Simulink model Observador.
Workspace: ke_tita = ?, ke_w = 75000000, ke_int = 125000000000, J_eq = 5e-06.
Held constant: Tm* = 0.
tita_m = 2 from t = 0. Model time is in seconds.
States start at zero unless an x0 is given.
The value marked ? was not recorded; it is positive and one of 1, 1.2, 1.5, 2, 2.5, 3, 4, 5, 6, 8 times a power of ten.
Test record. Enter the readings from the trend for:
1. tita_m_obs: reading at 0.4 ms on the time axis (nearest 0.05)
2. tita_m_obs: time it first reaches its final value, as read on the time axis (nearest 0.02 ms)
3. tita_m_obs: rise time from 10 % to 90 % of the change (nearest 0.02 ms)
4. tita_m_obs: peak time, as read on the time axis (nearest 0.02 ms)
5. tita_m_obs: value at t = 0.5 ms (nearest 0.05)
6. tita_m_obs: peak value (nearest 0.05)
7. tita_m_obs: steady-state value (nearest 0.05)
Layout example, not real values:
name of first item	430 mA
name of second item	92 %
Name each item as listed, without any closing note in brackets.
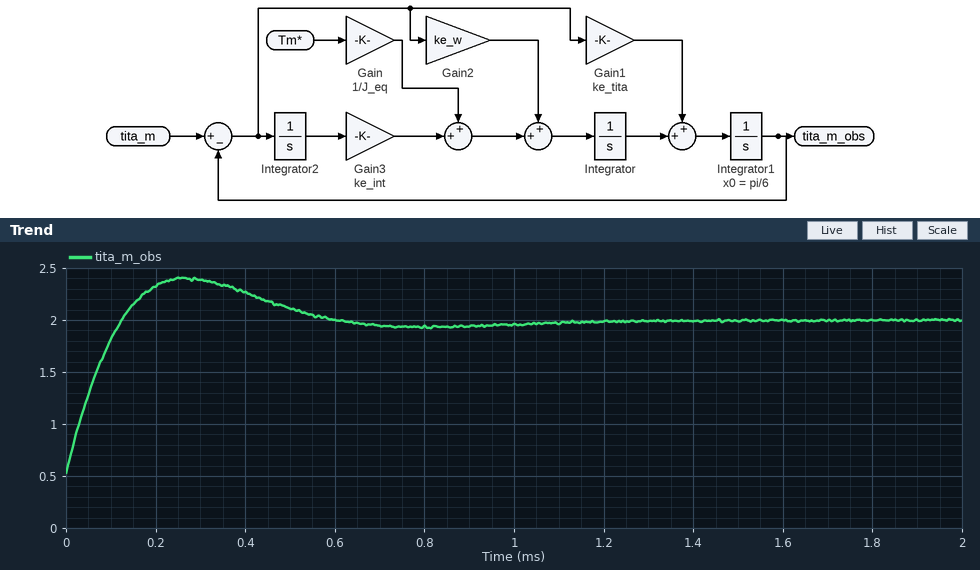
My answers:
tita_m_obs: reading at 0.4 ms on the time axis	2.25
tita_m_obs: time it first reaches its final value, as read on the time axis	0.12 ms
tita_m_obs: rise time from 10 % to 90 % of the change	0.10 ms
tita_m_obs: peak time, as read on the time axis	0.26 ms
tita_m_obs: value at t = 0.5 ms	2.10
tita_m_obs: peak value	2.40
tita_m_obs: steady-state value	2.00
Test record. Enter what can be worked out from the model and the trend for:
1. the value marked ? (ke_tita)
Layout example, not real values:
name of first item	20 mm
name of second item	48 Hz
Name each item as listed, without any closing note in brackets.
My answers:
the value marked ?	12000
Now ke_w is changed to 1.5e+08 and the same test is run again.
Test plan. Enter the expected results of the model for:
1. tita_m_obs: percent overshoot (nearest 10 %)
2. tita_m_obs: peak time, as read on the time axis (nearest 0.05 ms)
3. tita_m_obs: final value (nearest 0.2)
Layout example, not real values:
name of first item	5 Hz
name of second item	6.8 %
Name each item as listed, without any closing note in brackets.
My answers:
tita_m_obs: percent overshoot	30 %
tita_m_obs: peak time, as read on the time axis	0.20 ms
tita_m_obs: final value	2.0
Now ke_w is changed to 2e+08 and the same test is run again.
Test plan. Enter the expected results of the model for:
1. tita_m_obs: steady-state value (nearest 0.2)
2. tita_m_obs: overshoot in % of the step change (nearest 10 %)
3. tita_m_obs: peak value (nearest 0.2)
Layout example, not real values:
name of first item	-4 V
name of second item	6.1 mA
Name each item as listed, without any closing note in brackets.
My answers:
tita_m_obs: steady-state value	2.0
tita_m_obs: overshoot in % of the step change	40 %
tita_m_obs: peak value	2.6
